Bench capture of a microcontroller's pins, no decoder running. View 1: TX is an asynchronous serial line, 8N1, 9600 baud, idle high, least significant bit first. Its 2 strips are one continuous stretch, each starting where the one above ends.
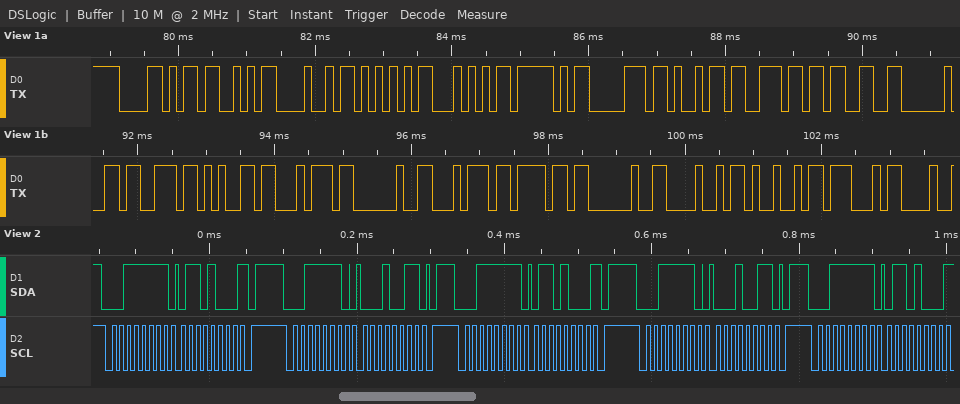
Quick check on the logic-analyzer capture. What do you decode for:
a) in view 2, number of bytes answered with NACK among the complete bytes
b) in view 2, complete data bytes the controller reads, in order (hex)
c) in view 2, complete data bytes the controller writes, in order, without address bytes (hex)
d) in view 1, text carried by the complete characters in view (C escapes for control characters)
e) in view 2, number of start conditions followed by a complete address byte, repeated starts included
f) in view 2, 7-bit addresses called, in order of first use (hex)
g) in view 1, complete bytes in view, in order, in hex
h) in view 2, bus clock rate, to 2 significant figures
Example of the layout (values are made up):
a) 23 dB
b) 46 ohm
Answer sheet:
a) 3
b) 68 68 68
c) 13 13
d) "XSHUT_pin3 set to HIG"
e) 5
f) 0x1F
g) 58 53 48 55 54 5F 70 69 6E 33 20 73 65 74 20 74 6F 20 48 49 47
h) 100 kHz
